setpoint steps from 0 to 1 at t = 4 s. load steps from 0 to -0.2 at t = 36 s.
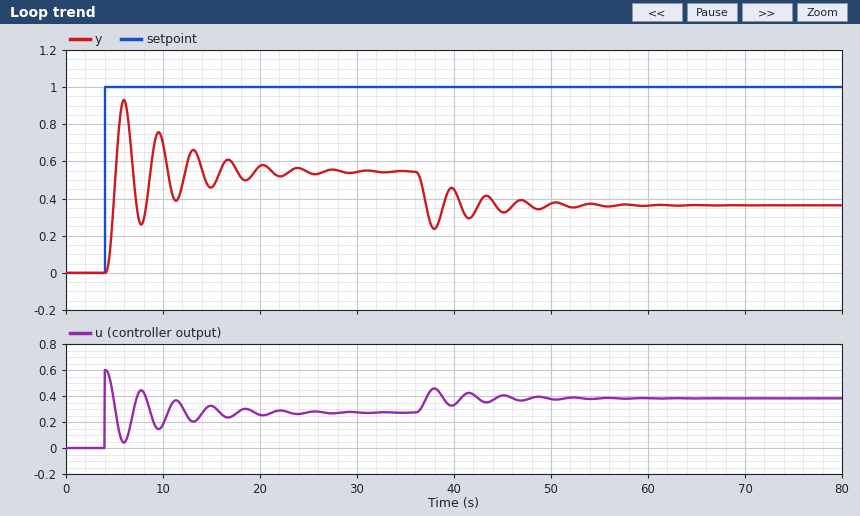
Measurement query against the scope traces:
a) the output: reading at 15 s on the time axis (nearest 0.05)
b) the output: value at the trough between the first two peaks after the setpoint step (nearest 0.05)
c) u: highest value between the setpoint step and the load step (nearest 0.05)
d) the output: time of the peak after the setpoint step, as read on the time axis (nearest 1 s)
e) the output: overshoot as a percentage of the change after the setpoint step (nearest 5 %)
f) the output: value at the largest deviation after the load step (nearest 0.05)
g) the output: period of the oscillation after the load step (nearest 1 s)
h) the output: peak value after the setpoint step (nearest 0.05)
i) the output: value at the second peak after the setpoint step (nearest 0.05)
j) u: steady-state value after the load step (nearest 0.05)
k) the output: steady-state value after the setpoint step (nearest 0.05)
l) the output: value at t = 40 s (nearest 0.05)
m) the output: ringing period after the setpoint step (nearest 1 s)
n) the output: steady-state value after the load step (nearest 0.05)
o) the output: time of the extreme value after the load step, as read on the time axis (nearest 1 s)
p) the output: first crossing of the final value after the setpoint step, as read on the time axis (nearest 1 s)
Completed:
0.45
0.25
0.60
6 s
70 %
0.25
4 s
0.95
0.75
0.40
0.55
0.45
4 s
0.35
38 s
5 s
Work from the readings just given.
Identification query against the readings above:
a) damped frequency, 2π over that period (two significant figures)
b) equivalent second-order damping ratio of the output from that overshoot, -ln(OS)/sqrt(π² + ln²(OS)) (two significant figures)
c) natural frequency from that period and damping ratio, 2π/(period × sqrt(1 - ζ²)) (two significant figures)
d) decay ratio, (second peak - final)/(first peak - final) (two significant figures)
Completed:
1.6 rad/s
0.11
1.6 rad/s
0.50
